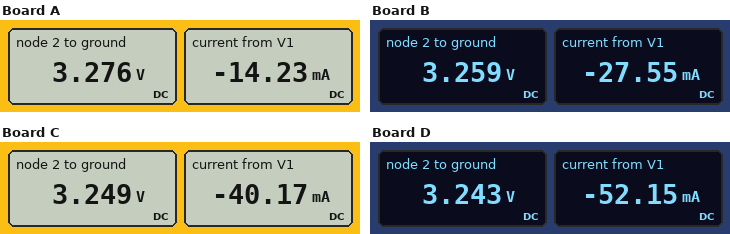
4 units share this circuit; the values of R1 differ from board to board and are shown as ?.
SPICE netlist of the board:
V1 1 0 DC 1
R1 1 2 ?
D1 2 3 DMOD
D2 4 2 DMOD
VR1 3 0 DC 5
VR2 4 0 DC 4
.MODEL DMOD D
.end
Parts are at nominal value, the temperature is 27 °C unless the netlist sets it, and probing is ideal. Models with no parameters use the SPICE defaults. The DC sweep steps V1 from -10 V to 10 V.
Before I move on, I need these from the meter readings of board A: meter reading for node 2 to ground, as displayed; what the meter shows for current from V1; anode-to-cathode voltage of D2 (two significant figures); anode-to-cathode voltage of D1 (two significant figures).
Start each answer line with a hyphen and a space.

- 3.276 V
- -14.23 mA
- 720 mV
- -1.7 V
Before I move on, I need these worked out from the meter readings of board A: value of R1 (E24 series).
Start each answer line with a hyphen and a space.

- 160 Ω
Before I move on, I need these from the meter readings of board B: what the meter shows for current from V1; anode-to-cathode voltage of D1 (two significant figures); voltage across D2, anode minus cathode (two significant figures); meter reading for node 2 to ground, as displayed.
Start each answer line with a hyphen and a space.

- -27.55 mA
- -1.7 V
- 740 mV
- 3.259 V
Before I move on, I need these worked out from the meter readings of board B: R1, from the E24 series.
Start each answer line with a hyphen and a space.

- 82 Ω
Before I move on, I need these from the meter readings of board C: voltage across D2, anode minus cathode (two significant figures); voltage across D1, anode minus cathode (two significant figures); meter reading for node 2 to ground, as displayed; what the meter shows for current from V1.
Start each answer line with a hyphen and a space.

- 750 mV
- -1.8 V
- 3.249 V
- -40.17 mA
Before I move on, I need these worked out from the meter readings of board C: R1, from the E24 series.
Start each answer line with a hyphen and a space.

- 56 Ω
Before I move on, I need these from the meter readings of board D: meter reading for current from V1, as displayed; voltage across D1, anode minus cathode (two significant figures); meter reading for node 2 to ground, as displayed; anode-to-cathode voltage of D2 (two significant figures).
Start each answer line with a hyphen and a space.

- -52.15 mA
- -1.8 V
- 3.243 V
- 760 mV
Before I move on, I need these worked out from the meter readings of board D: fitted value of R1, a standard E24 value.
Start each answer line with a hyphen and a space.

- 43 Ω
